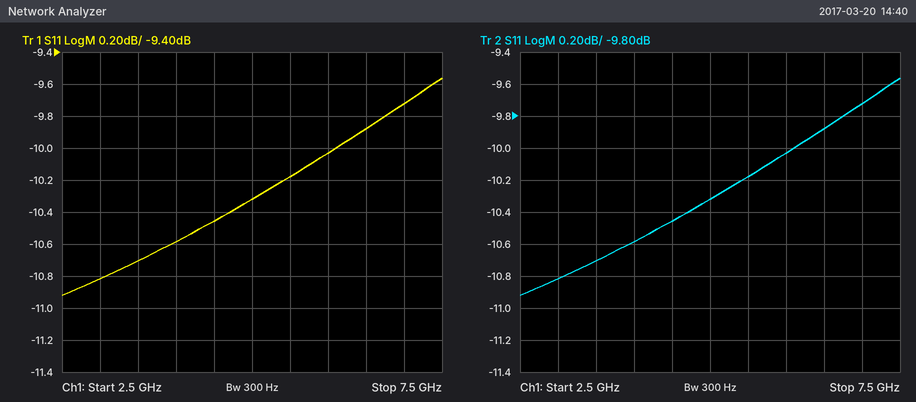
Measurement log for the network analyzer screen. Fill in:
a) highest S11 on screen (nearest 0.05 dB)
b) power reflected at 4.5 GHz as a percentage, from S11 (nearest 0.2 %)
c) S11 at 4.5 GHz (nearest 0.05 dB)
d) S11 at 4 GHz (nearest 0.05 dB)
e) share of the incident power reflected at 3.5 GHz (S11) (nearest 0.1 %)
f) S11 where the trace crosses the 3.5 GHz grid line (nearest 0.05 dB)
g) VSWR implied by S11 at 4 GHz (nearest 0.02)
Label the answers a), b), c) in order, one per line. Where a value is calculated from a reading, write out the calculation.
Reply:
a) -9.55 dB
b) 10^(-10.45/10) ≈ 9.0 %
c) -10.45 dB
d) -10.60 dB
e) 10^(-10.7/10) ≈ 8.5 %
f) -10.70 dB
g) |Γ| = 10^(-10.6/20) = 0.2951; VSWR = (1 + 0.2951)/(1 − 0.2951) ≈ 1.84
